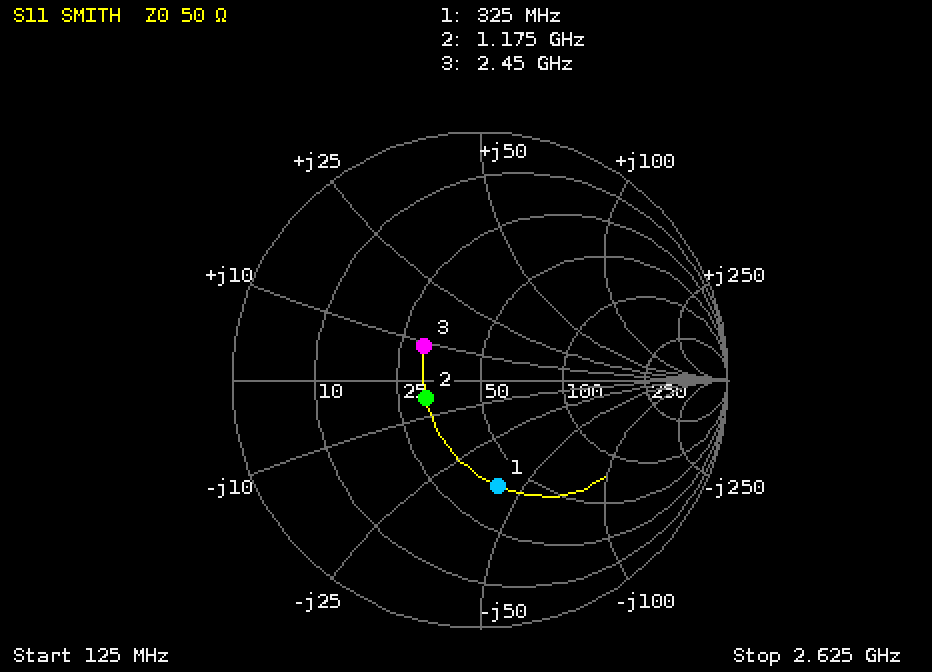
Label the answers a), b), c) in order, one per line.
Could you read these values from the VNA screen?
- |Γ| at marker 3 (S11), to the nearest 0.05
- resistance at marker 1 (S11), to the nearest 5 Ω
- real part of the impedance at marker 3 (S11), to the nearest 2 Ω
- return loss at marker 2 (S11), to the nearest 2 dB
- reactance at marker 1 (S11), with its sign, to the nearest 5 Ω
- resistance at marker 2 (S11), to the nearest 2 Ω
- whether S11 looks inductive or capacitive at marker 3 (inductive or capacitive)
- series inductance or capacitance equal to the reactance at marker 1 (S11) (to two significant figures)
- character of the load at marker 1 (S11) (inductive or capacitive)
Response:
a) 0.25
b) 40 Ω
c) 30 Ω
d) 12 dB
e) -40 Ω
f) 32 Ω
g) inductive
h) 12 pF
i) capacitive
